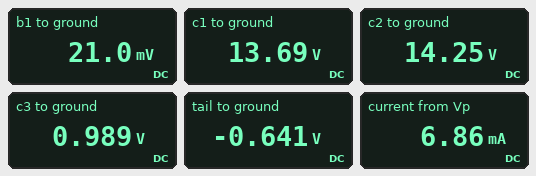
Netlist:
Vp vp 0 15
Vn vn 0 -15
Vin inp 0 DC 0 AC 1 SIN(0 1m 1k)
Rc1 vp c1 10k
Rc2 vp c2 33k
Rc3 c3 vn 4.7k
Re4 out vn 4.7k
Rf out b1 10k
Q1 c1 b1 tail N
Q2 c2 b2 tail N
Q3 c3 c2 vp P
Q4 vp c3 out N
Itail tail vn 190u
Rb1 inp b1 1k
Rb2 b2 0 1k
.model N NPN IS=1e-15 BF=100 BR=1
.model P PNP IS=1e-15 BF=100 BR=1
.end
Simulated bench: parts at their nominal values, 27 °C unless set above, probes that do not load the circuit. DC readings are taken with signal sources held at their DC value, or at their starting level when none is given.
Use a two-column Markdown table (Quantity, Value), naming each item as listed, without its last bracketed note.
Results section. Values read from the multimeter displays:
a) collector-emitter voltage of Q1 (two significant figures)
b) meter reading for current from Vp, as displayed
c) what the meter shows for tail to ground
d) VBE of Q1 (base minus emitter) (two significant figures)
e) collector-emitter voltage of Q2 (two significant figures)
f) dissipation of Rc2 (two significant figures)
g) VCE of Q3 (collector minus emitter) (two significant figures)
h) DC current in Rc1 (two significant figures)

| Quantity | Value |
|---|---|
| collector-emitter voltage of Q1 | 14 V |
| meter reading for current from Vp, as displayed | 6.86 mA |
| what the meter shows for tail to ground | -0.641 V |
| VBE of Q1 (base minus emitter) | 660 mV |
| collector-emitter voltage of Q2 | 15 V |
| dissipation of Rc2 | 17 µW |
| VCE of Q3 (collector minus emitter) | -14 V |
| DC current in Rc1 | 130 µA |
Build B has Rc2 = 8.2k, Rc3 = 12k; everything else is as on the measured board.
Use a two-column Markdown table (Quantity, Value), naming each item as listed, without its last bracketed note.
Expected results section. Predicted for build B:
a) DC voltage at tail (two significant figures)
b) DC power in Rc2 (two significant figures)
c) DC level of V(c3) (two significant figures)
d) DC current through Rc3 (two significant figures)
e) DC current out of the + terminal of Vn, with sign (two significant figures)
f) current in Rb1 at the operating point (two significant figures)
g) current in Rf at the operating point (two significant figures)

| Quantity | Value |
|---|---|
| DC voltage at tail | -660 mV |
| DC power in Rc2 | 64 µW |
| DC level of V(c3) | 700 mV |
| DC current through Rc3 | 1.3 mA |
| DC current out of the + terminal of Vn, with sign | -4.7 mA |
| current in Rb1 at the operating point | 5.1 µA |
| current in Rf at the operating point | 4.2 µA |
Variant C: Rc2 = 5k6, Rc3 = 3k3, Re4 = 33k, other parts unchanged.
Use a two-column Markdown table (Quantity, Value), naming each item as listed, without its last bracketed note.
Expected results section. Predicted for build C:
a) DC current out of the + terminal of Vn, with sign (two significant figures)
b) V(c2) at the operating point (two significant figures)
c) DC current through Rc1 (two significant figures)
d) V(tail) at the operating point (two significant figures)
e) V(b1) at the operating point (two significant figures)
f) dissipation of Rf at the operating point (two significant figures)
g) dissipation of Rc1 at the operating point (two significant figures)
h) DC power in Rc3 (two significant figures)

| Quantity | Value |
|---|---|
| DC current out of the + terminal of Vn, with sign | -5.1 mA |
| V(c2) at the operating point | 14 V |
| DC current through Rc1 | 8.7 µA |
| V(tail) at the operating point | -670 mV |
| V(b1) at the operating point | -80 mV |
| dissipation of Rf at the operating point | 64 µW |
| dissipation of Rc1 at the operating point | 750 nW |
| DC power in Rc3 | 66 mW |
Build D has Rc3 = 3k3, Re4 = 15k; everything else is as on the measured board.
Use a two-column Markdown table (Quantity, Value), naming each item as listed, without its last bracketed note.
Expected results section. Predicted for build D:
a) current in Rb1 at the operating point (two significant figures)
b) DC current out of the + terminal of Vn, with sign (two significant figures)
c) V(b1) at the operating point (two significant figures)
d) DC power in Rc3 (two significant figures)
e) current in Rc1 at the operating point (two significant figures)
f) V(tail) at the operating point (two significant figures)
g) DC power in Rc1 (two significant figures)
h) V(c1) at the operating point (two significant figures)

| Quantity | Value |
|---|---|
| current in Rb1 at the operating point | 12 µA |
| DC current out of the + terminal of Vn, with sign | -6.0 mA |
| V(b1) at the operating point | 12 mV |
| DC power in Rc3 | 76 mW |
| current in Rc1 at the operating point | 120 µA |
| V(tail) at the operating point | -650 mV |
| DC power in Rc1 | 140 µW |
| V(c1) at the operating point | 14 V |
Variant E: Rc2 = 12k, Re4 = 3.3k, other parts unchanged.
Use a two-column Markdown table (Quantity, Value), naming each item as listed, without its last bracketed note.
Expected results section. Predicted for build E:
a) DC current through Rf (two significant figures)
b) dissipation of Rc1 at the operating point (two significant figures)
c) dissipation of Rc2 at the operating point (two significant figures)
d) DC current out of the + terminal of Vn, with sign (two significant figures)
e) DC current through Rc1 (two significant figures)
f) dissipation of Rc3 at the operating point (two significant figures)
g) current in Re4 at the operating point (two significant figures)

| Quantity | Value |
|---|---|
| DC current through Rf | 1.2 µA |
| dissipation of Rc1 at the operating point | 85 µW |
| dissipation of Rc2 at the operating point | 46 µW |
| DC current out of the + terminal of Vn, with sign | -8.1 mA |
| DC current through Rc1 | 92 µA |
| dissipation of Rc3 at the operating point | 53 mW |
| current in Re4 at the operating point | 4.5 mA |
